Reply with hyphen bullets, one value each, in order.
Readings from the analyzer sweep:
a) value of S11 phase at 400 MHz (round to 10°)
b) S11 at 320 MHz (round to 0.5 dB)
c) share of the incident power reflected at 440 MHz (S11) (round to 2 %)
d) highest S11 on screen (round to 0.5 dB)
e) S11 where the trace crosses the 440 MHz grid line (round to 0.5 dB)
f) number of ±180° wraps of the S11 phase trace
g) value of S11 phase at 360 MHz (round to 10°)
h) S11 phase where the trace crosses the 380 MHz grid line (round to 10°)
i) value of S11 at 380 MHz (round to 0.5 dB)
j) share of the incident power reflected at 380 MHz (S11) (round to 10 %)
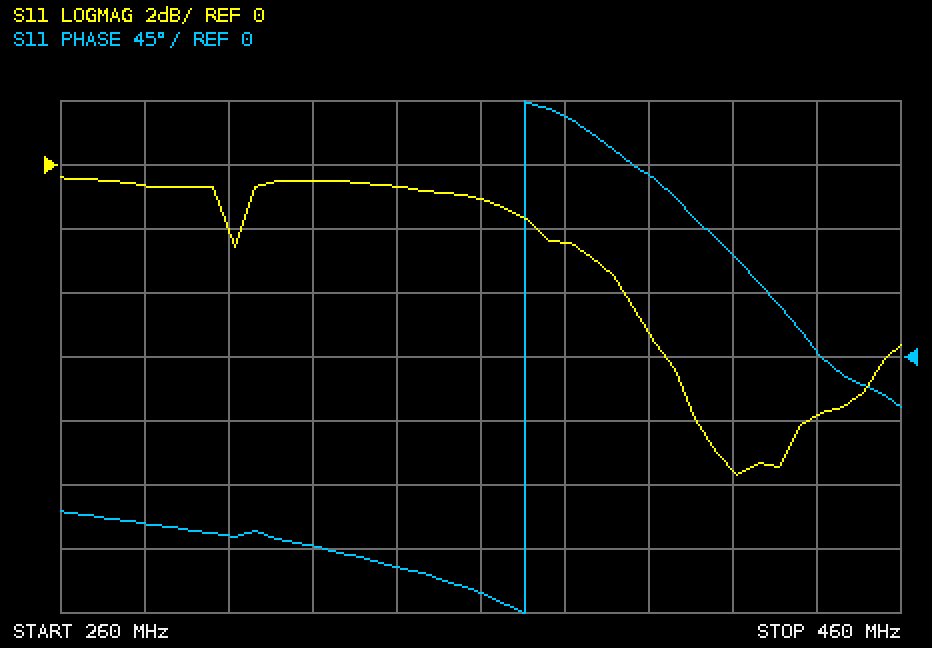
- 130°
- -0.5 dB
- 16 %
- -0.5 dB
- -8.0 dB
- 1
- -170°
- 170°
- -2.5 dB
- 60 %
